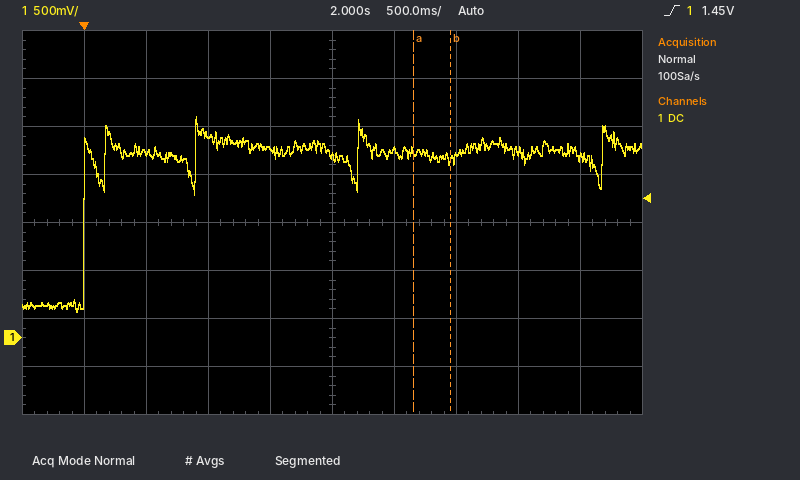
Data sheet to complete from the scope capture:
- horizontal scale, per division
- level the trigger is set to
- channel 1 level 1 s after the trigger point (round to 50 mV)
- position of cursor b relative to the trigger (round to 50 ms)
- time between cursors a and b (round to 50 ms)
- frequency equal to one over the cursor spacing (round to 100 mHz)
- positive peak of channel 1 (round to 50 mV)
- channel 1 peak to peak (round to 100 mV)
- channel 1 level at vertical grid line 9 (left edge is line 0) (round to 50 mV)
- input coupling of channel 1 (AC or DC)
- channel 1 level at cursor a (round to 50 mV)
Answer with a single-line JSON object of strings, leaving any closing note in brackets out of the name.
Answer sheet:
{"horizontal scale, per division": "500 ms", "level the trigger is set to": "1.45 V", "channel 1 level 1 s after the trigger point": "2.10 V", "position of cursor b relative to the trigger": "+2.95 s", "time between cursors a and b": "300 ms", "frequency equal to one over the cursor spacing": "3.3 Hz", "positive peak of channel 1": "2.30 V", "channel 1 peak to peak": "2.00 V", "channel 1 level at vertical grid line 9 (left edge is line 0)": "1.90 V", "input coupling of channel 1": "DC", "channel 1 level at cursor a": "1.95 V"}
